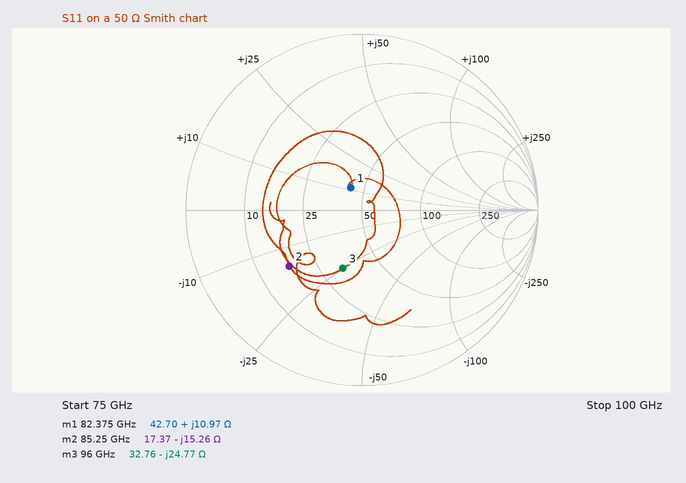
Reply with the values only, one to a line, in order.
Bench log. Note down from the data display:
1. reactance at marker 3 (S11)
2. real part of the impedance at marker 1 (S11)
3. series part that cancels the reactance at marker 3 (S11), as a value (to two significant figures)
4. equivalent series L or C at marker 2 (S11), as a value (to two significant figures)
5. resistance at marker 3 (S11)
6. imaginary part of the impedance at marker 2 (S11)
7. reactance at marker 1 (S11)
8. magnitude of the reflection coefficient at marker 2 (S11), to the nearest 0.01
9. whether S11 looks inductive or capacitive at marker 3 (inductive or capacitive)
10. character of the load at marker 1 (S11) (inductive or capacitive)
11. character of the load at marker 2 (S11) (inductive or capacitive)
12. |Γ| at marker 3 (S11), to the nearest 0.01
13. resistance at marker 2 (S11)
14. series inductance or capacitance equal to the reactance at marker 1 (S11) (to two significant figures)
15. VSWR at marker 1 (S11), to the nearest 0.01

-24.77 Ω
42.70 Ω
41 pH
120 fF
32.76 Ω
-15.26 Ω
+10.97 Ω
0.52
capacitive
inductive
capacitive
0.35
17.37 Ω
21 pH
1.33
